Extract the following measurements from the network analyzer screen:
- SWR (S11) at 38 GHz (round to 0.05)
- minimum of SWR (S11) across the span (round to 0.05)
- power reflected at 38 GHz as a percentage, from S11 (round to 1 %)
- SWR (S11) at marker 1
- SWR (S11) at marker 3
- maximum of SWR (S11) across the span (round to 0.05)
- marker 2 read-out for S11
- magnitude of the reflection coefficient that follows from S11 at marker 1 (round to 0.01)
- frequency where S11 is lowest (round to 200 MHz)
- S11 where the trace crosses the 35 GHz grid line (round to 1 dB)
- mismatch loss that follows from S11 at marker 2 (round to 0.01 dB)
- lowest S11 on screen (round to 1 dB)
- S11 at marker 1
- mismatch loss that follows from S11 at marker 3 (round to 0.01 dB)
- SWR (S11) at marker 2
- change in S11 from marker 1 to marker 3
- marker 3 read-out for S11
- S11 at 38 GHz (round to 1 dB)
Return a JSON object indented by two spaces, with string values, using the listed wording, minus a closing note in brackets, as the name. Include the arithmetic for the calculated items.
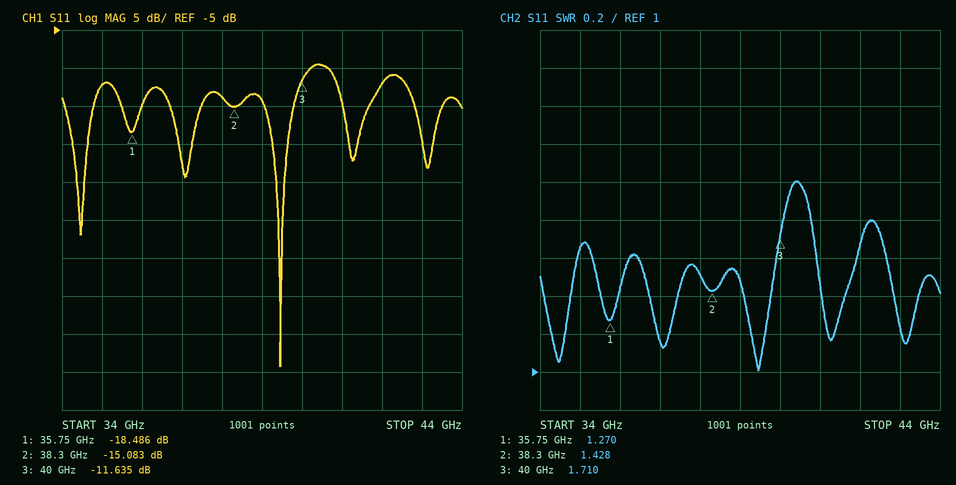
{
  "SWR (S11) at 38 GHz": "1.50",
  "minimum of SWR (S11) across the span": "1.00",
  "power reflected at 38 GHz as a percentage, from S11": "10^(-14/10) ≈ 4 %",
  "SWR (S11) at marker 1": "1.270",
  "SWR (S11) at marker 3": "1.710",
  "maximum of SWR (S11) across the span": "2.00",
  "marker 2 read-out for S11": "-15.083 dB",
  "magnitude of the reflection coefficient that follows from S11 at marker 1": "10^(-18.486/20) ≈ 0.12",
  "frequency where S11 is lowest": "39.4 GHz",
  "S11 where the trace crosses the 35 GHz grid line": "-12 dB",
  "mismatch loss that follows from S11 at marker 2": "−10 log10(1 − 10^(-15.083/10)) ≈ 0.14 dB",
  "lowest S11 on screen": "-49 dB",
  "S11 at marker 1": "-18.486 dB",
  "mismatch loss that follows from S11 at marker 3": "−10 log10(1 − 10^(-11.635/10)) ≈ 0.31 dB",
  "SWR (S11) at marker 2": "1.428",
  "change in S11 from marker 1 to marker 3": "-11.635 − (-18.486) = 6.851 dB",
  "marker 3 read-out for S11": "-11.635 dB",
  "S11 at 38 GHz": "-14 dB"
}
